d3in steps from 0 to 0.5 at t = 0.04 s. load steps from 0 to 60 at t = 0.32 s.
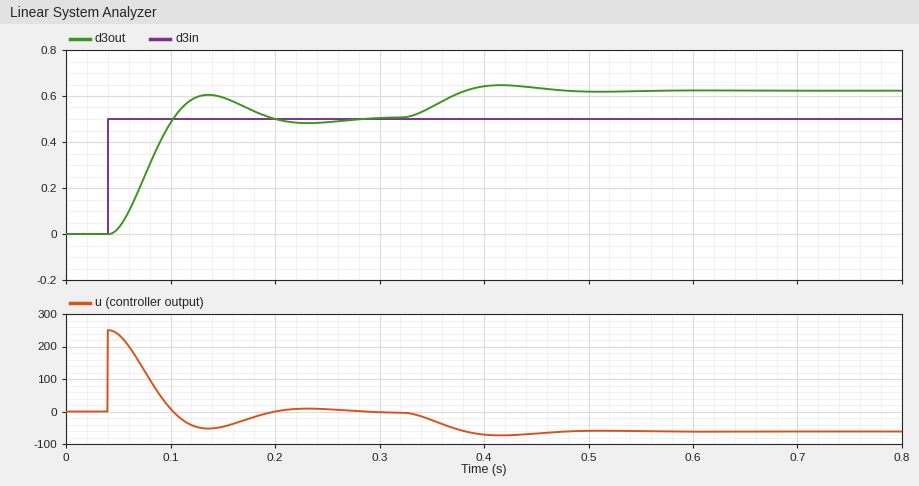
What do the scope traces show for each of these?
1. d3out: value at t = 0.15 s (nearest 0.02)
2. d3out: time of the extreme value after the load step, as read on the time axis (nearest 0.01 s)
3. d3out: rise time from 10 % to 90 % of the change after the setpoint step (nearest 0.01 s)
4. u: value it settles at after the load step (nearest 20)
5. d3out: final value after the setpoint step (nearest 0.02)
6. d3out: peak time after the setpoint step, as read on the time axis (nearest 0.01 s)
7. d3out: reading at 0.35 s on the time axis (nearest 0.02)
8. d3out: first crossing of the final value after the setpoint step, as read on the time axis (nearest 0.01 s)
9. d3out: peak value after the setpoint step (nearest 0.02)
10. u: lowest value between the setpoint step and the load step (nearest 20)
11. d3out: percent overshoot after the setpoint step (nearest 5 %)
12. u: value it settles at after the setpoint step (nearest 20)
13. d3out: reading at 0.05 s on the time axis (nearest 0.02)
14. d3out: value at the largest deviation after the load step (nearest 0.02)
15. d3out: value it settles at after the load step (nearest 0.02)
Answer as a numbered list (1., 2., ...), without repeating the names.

1. 0.60
2. 0.42 s
3. 0.04 s
4. -60
5. 0.50
6. 0.14 s
7. 0.56
8. 0.10 s
9. 0.60
10. -60
11. 20 %
12. 0
13. 0.02
14. 0.64
15. 0.62
